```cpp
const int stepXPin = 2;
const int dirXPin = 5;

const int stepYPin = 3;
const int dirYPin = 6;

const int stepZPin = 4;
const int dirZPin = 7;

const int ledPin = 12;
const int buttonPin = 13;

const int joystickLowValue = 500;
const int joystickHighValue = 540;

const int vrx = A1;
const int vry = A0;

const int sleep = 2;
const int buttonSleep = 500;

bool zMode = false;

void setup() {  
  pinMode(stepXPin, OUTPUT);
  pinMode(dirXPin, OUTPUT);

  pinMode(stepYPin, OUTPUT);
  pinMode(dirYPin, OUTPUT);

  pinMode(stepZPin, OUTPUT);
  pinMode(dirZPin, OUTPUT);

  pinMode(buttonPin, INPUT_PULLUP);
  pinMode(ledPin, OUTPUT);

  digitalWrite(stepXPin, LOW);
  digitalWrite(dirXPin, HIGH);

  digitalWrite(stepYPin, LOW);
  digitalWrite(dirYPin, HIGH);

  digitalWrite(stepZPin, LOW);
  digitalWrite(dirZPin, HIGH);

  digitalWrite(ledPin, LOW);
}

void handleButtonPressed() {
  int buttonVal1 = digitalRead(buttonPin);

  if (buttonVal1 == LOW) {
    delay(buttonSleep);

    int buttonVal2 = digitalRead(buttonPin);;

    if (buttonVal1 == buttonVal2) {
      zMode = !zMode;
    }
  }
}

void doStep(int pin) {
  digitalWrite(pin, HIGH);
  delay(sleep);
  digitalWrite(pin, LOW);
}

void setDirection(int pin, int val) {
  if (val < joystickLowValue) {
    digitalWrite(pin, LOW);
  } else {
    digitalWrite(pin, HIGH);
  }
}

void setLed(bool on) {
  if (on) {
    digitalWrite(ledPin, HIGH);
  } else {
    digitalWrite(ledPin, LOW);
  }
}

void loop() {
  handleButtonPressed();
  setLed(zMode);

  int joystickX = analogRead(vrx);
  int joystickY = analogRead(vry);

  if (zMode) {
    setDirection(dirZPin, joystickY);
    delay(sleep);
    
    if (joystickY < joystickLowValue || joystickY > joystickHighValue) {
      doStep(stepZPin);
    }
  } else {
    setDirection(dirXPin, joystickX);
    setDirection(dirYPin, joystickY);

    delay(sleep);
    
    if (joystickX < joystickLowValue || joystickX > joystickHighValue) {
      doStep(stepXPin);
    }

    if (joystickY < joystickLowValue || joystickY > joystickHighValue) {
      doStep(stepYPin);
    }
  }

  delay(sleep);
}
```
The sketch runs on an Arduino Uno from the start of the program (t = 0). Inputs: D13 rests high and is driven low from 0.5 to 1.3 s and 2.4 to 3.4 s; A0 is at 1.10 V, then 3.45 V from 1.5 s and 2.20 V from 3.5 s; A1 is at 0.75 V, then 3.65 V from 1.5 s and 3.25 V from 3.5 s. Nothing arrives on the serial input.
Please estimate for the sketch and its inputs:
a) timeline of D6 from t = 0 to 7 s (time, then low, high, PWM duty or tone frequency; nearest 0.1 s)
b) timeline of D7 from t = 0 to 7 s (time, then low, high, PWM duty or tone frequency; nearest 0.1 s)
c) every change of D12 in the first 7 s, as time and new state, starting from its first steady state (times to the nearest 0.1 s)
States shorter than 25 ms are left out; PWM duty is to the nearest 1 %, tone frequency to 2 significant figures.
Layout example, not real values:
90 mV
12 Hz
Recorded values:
0 s low; 2.9 s high; 3.5 s low
0 s high; 1 s low; 1.5 s high
0 s low; 1 s high; 2.9 s low
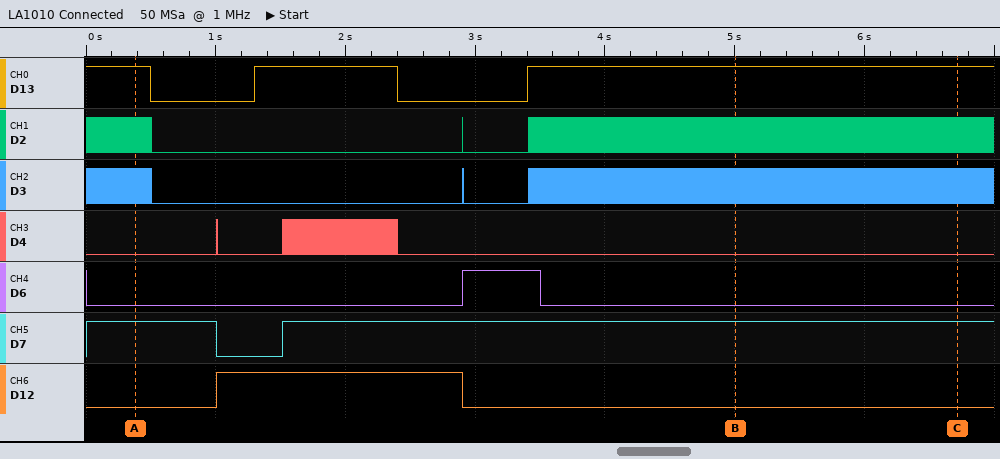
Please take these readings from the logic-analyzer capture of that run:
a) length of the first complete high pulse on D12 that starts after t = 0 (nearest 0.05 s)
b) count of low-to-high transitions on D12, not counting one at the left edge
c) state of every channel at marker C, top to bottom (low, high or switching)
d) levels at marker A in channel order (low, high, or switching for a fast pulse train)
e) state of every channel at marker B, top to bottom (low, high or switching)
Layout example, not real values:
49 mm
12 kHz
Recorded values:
1.90 s
1
D13 high, D2 switching, D3 switching, D4 low, D6 low, D7 high, D12 low
D13 high, D2 switching, D3 switching, D4 low, D6 low, D7 high, D12 low
D13 high, D2 switching, D3 switching, D4 low, D6 low, D7 high, D12 low
